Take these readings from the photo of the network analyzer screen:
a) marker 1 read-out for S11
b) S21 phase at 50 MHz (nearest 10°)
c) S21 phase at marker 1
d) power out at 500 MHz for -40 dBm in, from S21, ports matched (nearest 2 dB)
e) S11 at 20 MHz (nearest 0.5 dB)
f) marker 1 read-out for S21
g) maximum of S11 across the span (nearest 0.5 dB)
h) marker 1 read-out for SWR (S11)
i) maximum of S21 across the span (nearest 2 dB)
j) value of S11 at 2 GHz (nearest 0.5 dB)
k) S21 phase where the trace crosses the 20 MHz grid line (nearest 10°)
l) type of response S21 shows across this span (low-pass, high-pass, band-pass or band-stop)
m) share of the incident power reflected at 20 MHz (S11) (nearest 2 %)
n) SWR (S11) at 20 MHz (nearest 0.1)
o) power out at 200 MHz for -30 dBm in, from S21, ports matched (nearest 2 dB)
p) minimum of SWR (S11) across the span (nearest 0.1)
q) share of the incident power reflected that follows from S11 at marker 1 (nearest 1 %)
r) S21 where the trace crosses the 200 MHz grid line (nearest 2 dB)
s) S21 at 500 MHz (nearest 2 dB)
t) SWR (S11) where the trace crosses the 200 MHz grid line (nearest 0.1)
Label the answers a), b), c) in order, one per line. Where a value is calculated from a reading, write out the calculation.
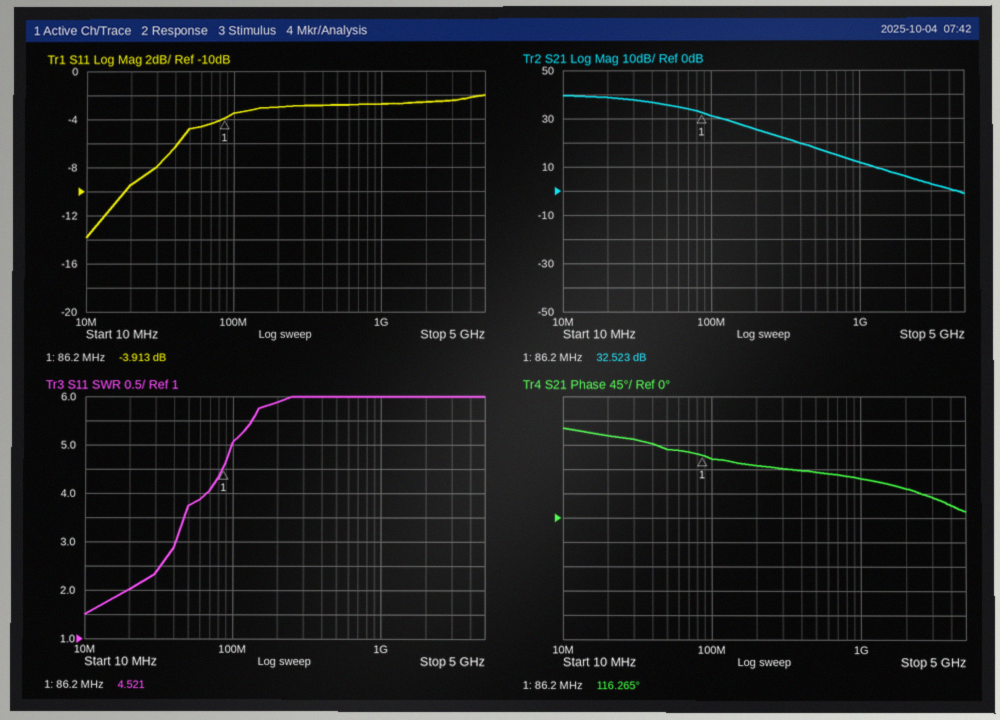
a) -3.913 dB
b) 130°
c) 116.265°
d) -40 dBm + (18 dB) = -22 dBm
e) -9.5 dB
f) 32.523 dB
g) -2.0 dB
h) 4.521
i) 40 dB
j) -2.5 dB
k) 150°
l) low-pass
m) 10^(-9.5/10) ≈ 11.2 %, so 12 % to the nearest 2 %
n) 2.0
o) -30 dBm + (26 dB) = -4 dBm
p) 1.5
q) 10^(-3.913/10) ≈ 41 %
r) 26 dB
s) 18 dB
t) 5.9
